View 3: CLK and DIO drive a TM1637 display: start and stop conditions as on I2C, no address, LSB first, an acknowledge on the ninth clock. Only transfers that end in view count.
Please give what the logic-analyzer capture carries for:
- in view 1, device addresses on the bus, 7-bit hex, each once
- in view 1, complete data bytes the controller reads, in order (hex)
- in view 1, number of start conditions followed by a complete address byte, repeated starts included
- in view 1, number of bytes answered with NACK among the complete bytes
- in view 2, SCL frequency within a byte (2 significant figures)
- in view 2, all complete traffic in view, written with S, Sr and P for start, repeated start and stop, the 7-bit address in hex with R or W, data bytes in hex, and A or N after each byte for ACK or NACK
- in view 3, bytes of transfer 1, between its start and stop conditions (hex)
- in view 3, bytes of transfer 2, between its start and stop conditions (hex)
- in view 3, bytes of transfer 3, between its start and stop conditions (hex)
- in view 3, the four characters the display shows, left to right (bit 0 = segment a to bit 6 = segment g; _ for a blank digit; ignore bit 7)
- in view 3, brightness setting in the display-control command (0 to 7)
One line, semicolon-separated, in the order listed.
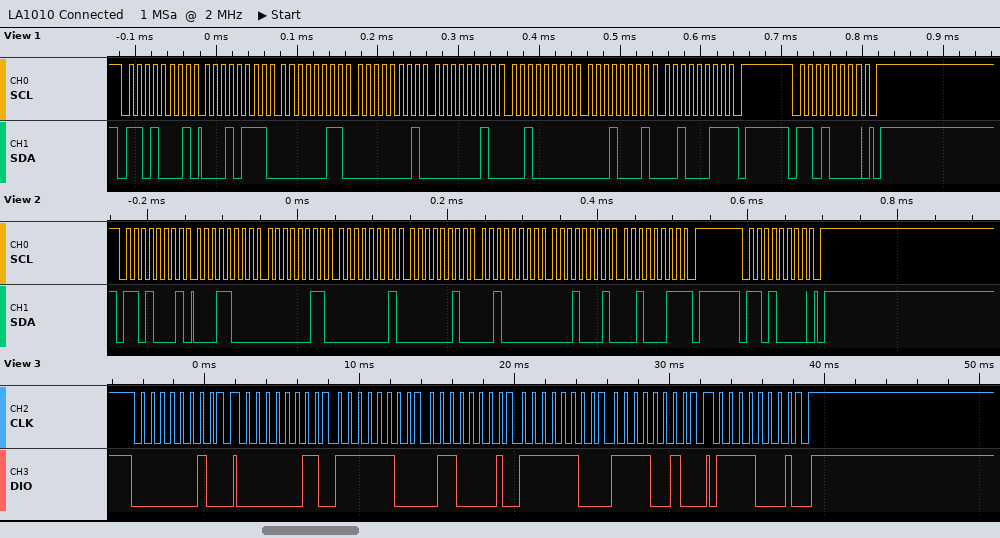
0x68; 17 03 01 02 20 11 23; 2; 1; 100 kHz; S 68R A 18 A 03 A 01 A 02 A 20 A 11 A 23 N P S 68W A P; 40; C0 3F 86 3F 4F; 8F; 0103; 7
